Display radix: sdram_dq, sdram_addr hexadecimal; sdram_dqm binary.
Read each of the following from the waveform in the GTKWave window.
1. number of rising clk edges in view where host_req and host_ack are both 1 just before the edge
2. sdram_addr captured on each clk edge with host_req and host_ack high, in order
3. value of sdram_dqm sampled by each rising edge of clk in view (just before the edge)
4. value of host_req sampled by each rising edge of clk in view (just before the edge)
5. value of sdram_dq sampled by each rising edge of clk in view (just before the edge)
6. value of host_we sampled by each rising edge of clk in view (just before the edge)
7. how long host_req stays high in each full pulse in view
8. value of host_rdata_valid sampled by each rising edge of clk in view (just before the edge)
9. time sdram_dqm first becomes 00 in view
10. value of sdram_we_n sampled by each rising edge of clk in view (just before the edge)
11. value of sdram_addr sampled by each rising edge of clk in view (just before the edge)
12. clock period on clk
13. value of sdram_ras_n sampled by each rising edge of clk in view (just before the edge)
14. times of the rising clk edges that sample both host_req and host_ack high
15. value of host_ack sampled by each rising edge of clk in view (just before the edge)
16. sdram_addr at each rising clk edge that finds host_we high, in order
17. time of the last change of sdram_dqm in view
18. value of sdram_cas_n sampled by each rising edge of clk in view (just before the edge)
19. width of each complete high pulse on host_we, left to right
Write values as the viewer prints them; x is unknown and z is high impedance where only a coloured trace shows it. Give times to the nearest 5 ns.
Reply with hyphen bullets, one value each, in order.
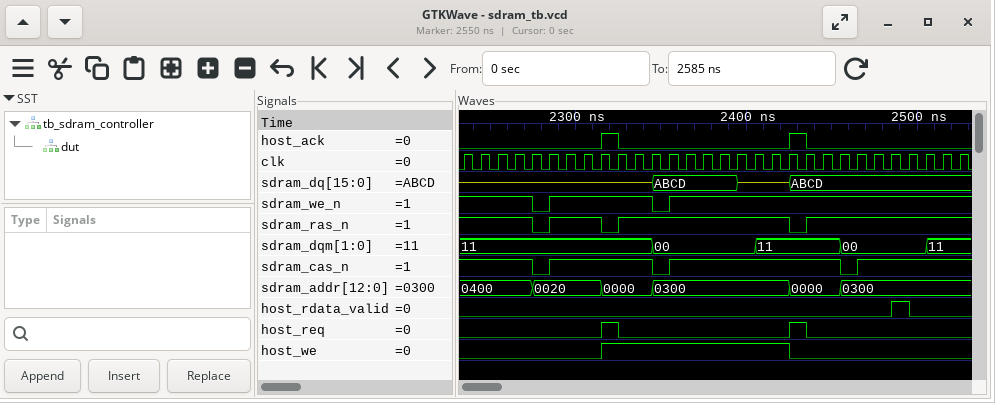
- 2
- 0000, 0000
- 11, 11, 11, 11, 11, 11, 11, 11, 11, 11, 11, 11, 00, 00, 00, 00, 00, 00, 11, 11, 11, 11, 11, 00, 00, 00, 00, 00, 11, 11
- 0 0 0 0 0 0 0 0 0 1 0 0 0 0 0 0 0 0 0 0 1 0 0 0 0 0 0 0 0 0
- z, z, z, z, z, z, z, z, z, z, z, z, ABCD, ABCD, ABCD, ABCD, ABCD, z, z, z, ABCD, ABCD, ABCD, ABCD, ABCD, ABCD, ABCD, ABCD, ABCD, ABCD
- 0 0 0 0 0 0 0 0 0 1 1 1 1 1 1 1 1 1 1 1 0 0 0 0 0 0 0 0 0 0
- 10 ns, 10 ns
- 0 0 0 0 0 0 0 0 0 0 0 0 0 0 0 0 0 0 0 0 0 0 0 0 0 0 1 0 0 0
- 2345 ns
- 1 1 1 1 1 0 1 1 1 1 1 1 0 1 1 1 1 1 1 1 1 1 1 1 1 1 1 1 1 1
- 0400, 0400, 0400, 0400, 0400, 0020, 0020, 0020, 0020, 0000, 0000, 0000, 0300, 0300, 0300, 0300, 0300, 0300, 0300, 0300, 0000, 0000, 0000, 0300, 0300, 0300, 0300, 0300, 0300, 0300
- 10 ns
- 1 1 1 1 1 0 1 1 1 0 1 1 1 1 1 1 1 1 1 1 0 1 1 1 1 1 1 1 1 1
- 2325 ns, 2435 ns
- 0 0 0 0 0 0 0 0 0 1 0 0 0 0 0 0 0 0 0 0 1 0 0 0 0 0 0 0 0 0
- 0000, 0000, 0000, 0300, 0300, 0300, 0300, 0300, 0300, 0300, 0300
- 2505 ns
- 1 1 1 1 1 0 1 1 1 1 1 1 0 1 1 1 1 1 1 1 1 1 1 0 1 1 1 1 1 1
- 110 ns
